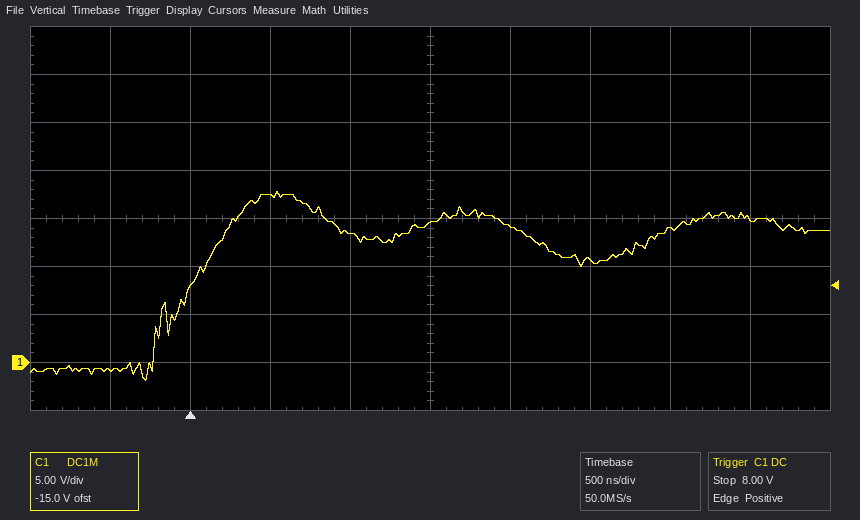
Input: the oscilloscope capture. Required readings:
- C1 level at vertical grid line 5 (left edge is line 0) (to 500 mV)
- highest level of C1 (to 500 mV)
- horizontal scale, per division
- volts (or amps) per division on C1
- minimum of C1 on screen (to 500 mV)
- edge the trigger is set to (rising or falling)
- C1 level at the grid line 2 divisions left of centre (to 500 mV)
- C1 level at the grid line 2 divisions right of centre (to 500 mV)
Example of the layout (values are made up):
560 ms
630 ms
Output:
14.5 V
18.0 V
500 ns
5 V
-2.0 V
rising
17.5 V
10.5 V
